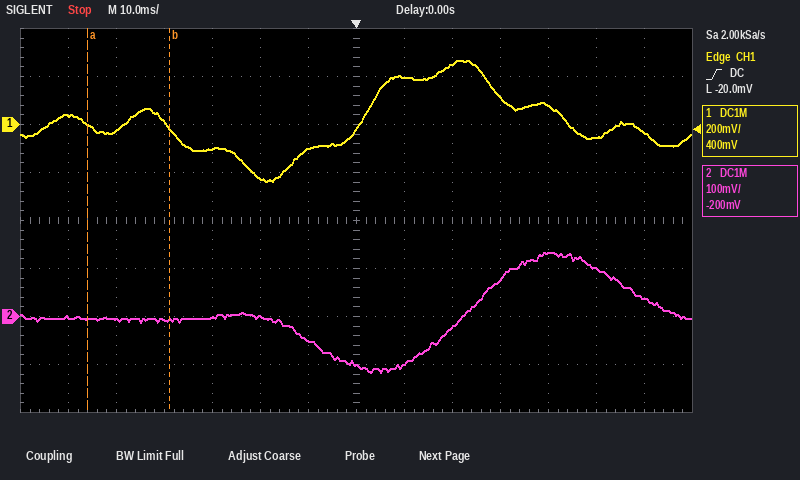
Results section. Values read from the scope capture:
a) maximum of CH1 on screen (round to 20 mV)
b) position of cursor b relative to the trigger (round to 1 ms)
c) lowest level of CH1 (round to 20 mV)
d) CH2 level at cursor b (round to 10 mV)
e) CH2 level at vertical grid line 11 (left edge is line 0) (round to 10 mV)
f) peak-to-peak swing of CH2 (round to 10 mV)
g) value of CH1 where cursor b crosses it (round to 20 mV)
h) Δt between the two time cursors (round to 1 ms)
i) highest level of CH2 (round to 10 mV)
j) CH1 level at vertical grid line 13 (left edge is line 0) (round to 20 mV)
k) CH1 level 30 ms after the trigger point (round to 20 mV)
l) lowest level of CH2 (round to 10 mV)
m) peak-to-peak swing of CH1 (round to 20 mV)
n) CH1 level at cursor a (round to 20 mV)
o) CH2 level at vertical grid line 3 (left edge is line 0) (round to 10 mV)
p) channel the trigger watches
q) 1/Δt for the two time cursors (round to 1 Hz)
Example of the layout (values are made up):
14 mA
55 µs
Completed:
260 mV
-39 ms
-240 mV
-10 mV
130 mV
250 mV
-20 mV
17 ms
130 mV
-40 mV
120 mV
-120 mV
500 mV
0 mV
-10 mV
CH1
59 Hz
